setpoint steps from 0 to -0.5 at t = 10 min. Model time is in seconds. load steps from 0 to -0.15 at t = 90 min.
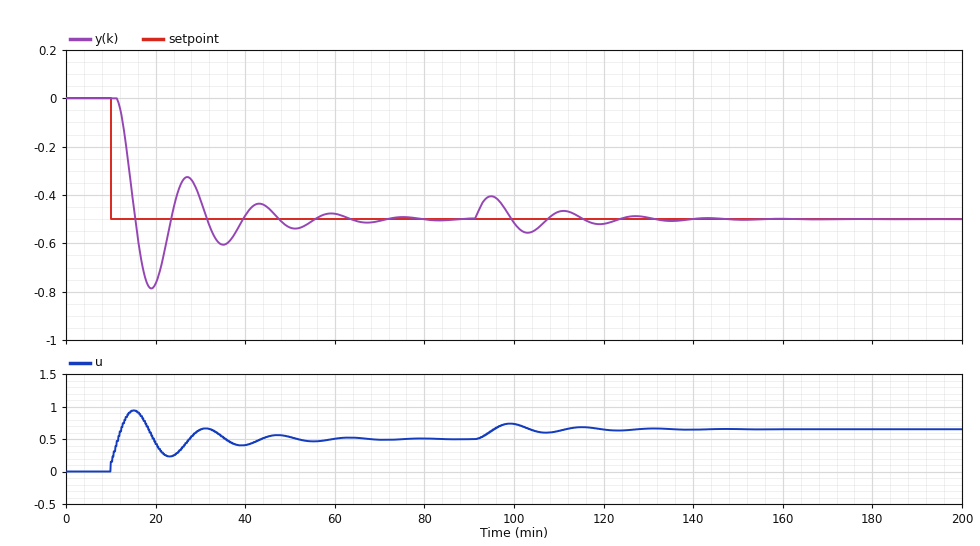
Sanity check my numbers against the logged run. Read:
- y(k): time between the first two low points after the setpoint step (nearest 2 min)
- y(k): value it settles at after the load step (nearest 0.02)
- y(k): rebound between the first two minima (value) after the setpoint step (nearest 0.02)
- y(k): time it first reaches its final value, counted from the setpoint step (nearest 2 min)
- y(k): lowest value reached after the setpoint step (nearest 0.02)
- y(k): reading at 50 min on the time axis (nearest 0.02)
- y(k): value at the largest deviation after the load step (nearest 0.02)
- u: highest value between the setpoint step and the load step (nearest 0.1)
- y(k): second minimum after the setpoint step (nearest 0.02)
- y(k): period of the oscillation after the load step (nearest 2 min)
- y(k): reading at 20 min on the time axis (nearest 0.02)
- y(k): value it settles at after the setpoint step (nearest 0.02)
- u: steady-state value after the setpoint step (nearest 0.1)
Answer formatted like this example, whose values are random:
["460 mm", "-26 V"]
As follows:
["16 min", "-0.50", "-0.32", "6 min", "-0.78", "-0.54", "-0.40", "0.9", "-0.60", "16 min", "-0.76", "-0.50", "0.5"]
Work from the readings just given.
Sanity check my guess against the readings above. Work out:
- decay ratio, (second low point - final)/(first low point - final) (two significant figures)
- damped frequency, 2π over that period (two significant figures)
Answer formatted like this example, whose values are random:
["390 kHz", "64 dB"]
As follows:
["0.36", "0.39 rad/min"]
